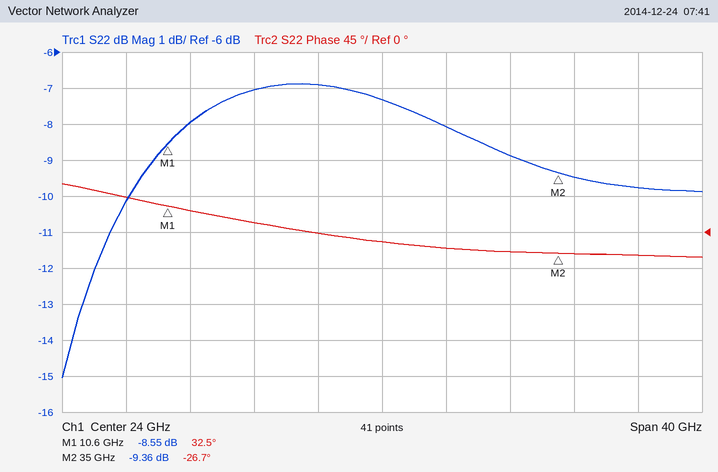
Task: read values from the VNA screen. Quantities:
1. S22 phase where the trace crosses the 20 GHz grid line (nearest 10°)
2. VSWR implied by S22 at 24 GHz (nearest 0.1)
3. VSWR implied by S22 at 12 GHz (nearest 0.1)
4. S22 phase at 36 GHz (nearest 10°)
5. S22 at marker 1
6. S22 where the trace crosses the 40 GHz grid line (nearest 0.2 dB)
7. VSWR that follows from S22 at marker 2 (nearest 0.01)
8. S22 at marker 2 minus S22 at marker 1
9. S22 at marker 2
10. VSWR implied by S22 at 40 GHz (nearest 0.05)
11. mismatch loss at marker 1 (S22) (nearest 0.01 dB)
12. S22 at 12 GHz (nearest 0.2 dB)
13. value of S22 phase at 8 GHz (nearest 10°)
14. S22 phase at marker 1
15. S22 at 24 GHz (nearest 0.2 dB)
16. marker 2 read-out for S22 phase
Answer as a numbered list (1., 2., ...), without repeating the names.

1. 0°
2. 2.5
3. 2.3
4. -30°
5. -8.55 dB
6. -9.8 dB
7. 2.03
8. -0.81 dB
9. -9.36 dB
10. 1.95
11. 0.65 dB
12. -8.0 dB
13. 40°
14. 32.5°
15. -7.4 dB
16. -26.7°
